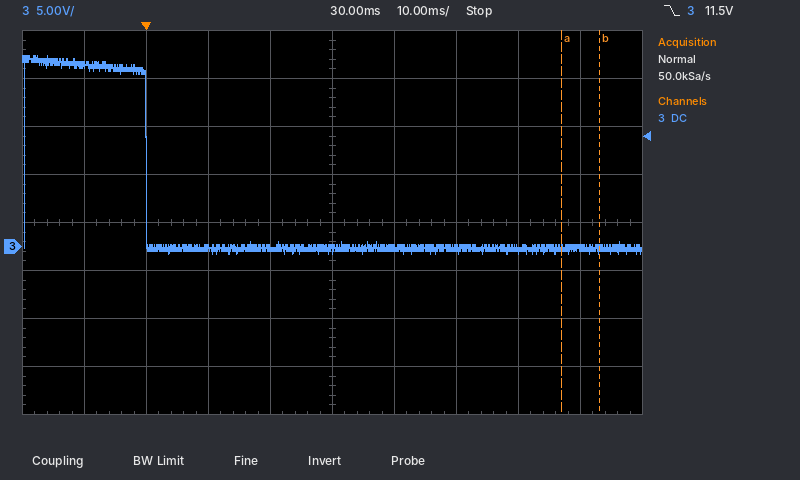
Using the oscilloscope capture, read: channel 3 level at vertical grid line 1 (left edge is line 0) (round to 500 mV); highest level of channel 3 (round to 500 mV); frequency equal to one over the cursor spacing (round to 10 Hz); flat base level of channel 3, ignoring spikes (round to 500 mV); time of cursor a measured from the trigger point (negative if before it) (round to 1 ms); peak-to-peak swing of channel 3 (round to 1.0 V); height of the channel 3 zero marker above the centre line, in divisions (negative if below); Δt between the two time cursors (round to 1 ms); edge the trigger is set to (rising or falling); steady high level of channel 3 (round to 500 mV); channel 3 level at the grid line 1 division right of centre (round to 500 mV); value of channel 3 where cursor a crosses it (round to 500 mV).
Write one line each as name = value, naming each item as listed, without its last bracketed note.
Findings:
channel 3 level at vertical grid line 1 (left edge is line 0) = 19.0 V
highest level of channel 3 = 20.0 V
frequency equal to one over the cursor spacing = 170 Hz
flat base level of channel 3, ignoring spikes = 0.0 V
time of cursor a measured from the trigger point (negative if before it) = +67 ms
peak-to-peak swing of channel 3 = 21.0 V
height of the channel 3 zero marker above the centre line, in divisions = -0.5 div
Δt between the two time cursors = 6 ms
edge the trigger is set to = falling
steady high level of channel 3 = 19.0 V
channel 3 level at the grid line 1 division right of centre = 0.0 V
value of channel 3 where cursor a crosses it = 0.0 V
